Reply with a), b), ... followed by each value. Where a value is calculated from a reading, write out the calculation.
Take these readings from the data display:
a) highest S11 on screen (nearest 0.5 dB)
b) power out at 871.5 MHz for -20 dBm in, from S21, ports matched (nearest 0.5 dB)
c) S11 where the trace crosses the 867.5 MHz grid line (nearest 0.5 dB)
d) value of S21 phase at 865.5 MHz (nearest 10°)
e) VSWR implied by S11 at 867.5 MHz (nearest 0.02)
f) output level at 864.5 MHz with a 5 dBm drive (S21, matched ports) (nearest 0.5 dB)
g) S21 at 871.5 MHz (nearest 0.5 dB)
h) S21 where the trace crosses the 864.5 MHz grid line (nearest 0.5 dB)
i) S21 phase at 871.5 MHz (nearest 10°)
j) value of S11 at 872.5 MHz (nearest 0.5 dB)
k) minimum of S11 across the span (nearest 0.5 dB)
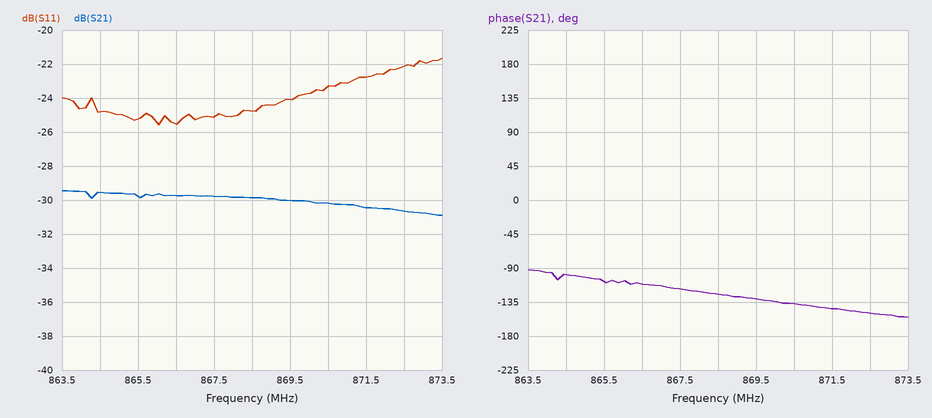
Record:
a) -21.5 dB
b) -20 dBm + (-30.5 dB) = -50.5 dBm
c) -25.0 dB
d) -110°
e) |Γ| = 10^(-25/20) = 0.0562; VSWR = (1 + 0.0562)/(1 − 0.0562) ≈ 1.12
f) 5 dBm + (-29.5 dB) = -24.5 dBm
g) -30.5 dB
h) -29.5 dB
i) -140°
j) -22.0 dB
k) -25.5 dB
